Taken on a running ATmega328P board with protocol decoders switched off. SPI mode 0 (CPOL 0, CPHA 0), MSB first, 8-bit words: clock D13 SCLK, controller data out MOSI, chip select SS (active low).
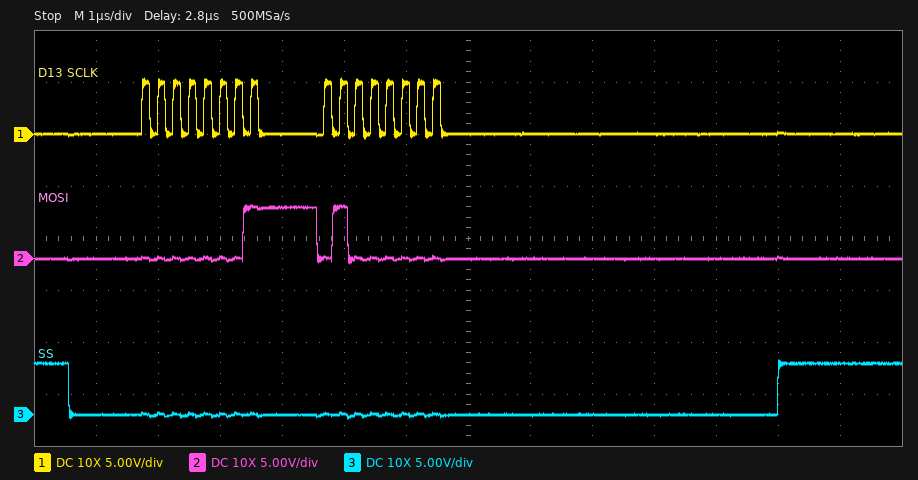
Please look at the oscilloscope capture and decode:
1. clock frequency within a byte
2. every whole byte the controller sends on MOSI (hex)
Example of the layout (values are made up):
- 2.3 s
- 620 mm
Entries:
- 4 MHz
- 01 40
